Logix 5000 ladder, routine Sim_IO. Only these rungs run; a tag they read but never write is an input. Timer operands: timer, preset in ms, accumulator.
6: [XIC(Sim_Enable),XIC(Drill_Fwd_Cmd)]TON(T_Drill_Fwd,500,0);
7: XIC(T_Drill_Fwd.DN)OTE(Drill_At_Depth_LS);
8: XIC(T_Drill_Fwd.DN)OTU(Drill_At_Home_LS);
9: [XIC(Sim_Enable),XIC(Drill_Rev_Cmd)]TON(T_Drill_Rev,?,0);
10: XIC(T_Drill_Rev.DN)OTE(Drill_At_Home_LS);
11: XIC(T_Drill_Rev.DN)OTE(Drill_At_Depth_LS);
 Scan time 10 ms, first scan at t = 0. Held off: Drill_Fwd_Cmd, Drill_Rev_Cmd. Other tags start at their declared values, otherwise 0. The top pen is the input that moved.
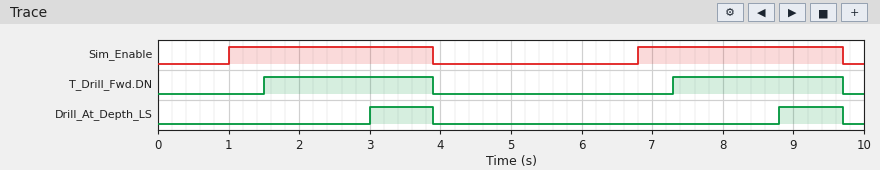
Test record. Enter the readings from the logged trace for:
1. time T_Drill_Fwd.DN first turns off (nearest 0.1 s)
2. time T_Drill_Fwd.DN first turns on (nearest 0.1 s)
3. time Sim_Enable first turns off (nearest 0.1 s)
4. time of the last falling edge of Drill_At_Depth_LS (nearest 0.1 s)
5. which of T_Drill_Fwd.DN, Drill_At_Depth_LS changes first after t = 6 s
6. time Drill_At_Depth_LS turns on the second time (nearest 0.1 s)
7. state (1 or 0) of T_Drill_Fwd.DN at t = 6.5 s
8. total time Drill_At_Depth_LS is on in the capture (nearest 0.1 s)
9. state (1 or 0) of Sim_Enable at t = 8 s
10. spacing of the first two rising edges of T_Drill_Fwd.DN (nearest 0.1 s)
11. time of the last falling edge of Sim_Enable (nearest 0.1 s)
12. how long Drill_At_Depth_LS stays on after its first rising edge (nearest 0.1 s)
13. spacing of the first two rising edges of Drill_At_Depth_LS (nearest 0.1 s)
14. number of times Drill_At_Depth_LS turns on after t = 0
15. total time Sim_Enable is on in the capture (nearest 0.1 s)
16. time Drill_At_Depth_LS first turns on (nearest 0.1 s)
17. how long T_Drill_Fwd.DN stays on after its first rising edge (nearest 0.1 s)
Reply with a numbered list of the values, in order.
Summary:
1. 3.9 s
2. 1.5 s
3. 3.9 s
4. 9.7 s
5. T_Drill_Fwd.DN
6. 8.8 s
7. 0
8. 1.8 s
9. 1
10. 5.8 s
11. 9.7 s
12. 0.9 s
13. 5.8 s
14. 2
15. 5.8 s
16. 3.0 s
17. 2.4 s
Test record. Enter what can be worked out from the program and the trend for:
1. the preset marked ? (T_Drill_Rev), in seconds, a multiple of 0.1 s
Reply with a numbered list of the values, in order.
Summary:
1. 2.0 s
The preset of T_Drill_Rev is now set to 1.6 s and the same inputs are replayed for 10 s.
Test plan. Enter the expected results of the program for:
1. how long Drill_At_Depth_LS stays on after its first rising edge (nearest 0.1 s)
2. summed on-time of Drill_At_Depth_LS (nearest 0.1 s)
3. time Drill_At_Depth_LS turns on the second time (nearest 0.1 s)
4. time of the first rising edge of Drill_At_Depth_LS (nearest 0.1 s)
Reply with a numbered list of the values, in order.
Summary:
1. 1.3 s
2. 2.6 s
3. 8.4 s
4. 2.6 s
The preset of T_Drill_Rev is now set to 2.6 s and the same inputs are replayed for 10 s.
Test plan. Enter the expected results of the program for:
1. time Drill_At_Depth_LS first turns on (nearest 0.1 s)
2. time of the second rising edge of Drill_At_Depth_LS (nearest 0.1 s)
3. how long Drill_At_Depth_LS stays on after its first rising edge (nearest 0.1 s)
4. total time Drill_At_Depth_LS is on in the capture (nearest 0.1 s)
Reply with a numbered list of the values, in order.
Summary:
1. 3.6 s
2. 9.4 s
3. 0.3 s
4. 0.6 s
